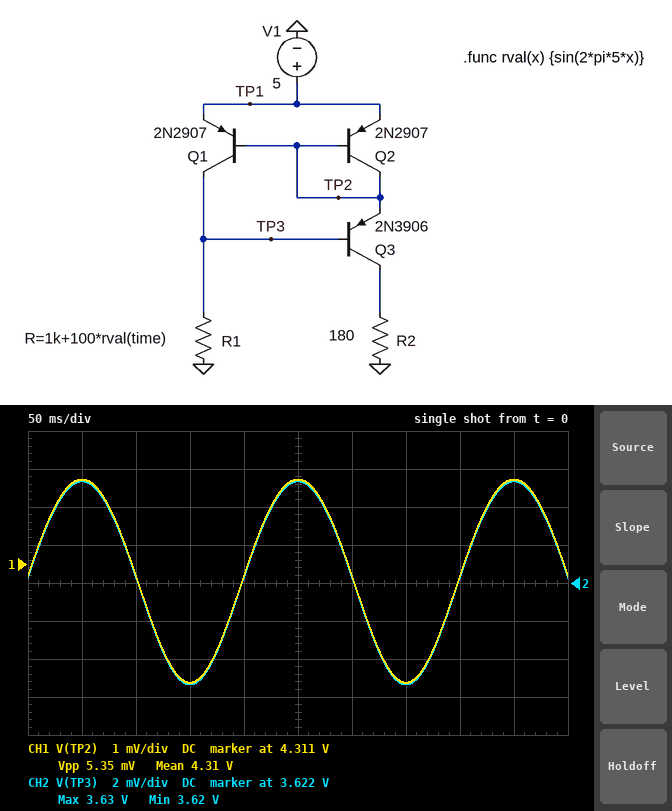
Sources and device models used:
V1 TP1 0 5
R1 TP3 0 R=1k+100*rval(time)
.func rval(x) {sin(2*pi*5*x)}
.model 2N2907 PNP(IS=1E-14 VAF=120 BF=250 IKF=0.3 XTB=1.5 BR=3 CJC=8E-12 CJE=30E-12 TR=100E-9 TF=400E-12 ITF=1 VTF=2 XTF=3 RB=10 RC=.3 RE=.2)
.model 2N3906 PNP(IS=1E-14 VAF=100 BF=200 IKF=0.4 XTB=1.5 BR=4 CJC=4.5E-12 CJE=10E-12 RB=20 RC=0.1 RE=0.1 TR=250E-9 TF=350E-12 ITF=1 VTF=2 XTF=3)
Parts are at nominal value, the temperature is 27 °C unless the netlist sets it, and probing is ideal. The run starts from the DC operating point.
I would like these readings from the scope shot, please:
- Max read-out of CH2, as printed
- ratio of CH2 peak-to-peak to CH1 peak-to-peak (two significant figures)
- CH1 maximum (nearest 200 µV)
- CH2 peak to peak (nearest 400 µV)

3.63 V
2.0
4.3132 V
10.8 mV
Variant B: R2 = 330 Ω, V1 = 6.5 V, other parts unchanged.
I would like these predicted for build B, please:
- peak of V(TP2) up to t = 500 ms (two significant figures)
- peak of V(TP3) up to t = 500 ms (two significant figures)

5.8 V
5.1 V
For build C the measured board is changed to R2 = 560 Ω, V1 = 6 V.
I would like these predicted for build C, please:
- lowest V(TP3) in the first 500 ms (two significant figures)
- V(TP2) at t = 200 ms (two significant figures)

4.6 V
5.3 V
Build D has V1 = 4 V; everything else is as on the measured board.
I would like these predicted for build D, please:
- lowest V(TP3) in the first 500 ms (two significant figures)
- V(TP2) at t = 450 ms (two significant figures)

2.6 V
3.3 V
